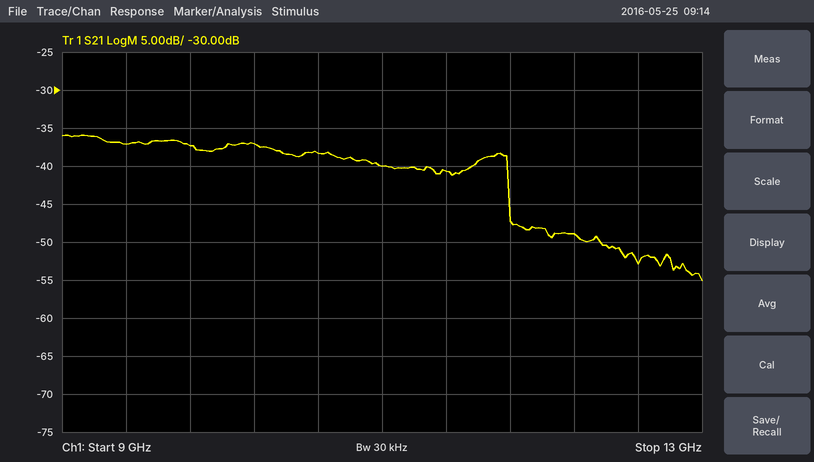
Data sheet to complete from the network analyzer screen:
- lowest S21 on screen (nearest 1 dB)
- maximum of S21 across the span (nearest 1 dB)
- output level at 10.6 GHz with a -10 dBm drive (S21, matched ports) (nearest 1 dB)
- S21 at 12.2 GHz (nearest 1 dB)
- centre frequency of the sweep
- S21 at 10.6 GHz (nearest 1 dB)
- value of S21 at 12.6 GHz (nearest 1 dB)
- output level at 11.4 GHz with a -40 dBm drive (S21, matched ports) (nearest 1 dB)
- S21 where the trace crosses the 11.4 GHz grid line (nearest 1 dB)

-55 dB
-36 dB
-48 dBm
-49 dB
11 GHz
-38 dB
-53 dB
-81 dBm
-41 dB
